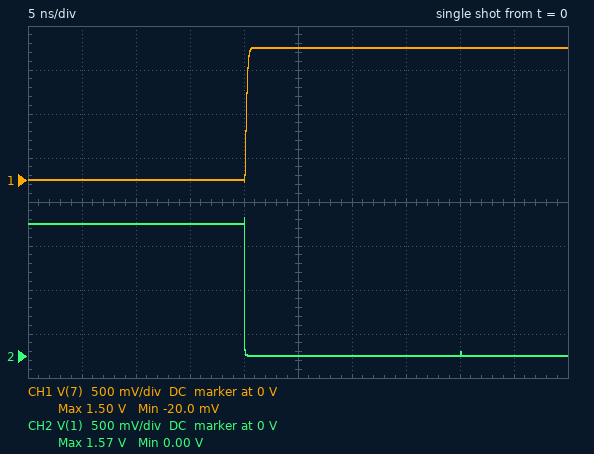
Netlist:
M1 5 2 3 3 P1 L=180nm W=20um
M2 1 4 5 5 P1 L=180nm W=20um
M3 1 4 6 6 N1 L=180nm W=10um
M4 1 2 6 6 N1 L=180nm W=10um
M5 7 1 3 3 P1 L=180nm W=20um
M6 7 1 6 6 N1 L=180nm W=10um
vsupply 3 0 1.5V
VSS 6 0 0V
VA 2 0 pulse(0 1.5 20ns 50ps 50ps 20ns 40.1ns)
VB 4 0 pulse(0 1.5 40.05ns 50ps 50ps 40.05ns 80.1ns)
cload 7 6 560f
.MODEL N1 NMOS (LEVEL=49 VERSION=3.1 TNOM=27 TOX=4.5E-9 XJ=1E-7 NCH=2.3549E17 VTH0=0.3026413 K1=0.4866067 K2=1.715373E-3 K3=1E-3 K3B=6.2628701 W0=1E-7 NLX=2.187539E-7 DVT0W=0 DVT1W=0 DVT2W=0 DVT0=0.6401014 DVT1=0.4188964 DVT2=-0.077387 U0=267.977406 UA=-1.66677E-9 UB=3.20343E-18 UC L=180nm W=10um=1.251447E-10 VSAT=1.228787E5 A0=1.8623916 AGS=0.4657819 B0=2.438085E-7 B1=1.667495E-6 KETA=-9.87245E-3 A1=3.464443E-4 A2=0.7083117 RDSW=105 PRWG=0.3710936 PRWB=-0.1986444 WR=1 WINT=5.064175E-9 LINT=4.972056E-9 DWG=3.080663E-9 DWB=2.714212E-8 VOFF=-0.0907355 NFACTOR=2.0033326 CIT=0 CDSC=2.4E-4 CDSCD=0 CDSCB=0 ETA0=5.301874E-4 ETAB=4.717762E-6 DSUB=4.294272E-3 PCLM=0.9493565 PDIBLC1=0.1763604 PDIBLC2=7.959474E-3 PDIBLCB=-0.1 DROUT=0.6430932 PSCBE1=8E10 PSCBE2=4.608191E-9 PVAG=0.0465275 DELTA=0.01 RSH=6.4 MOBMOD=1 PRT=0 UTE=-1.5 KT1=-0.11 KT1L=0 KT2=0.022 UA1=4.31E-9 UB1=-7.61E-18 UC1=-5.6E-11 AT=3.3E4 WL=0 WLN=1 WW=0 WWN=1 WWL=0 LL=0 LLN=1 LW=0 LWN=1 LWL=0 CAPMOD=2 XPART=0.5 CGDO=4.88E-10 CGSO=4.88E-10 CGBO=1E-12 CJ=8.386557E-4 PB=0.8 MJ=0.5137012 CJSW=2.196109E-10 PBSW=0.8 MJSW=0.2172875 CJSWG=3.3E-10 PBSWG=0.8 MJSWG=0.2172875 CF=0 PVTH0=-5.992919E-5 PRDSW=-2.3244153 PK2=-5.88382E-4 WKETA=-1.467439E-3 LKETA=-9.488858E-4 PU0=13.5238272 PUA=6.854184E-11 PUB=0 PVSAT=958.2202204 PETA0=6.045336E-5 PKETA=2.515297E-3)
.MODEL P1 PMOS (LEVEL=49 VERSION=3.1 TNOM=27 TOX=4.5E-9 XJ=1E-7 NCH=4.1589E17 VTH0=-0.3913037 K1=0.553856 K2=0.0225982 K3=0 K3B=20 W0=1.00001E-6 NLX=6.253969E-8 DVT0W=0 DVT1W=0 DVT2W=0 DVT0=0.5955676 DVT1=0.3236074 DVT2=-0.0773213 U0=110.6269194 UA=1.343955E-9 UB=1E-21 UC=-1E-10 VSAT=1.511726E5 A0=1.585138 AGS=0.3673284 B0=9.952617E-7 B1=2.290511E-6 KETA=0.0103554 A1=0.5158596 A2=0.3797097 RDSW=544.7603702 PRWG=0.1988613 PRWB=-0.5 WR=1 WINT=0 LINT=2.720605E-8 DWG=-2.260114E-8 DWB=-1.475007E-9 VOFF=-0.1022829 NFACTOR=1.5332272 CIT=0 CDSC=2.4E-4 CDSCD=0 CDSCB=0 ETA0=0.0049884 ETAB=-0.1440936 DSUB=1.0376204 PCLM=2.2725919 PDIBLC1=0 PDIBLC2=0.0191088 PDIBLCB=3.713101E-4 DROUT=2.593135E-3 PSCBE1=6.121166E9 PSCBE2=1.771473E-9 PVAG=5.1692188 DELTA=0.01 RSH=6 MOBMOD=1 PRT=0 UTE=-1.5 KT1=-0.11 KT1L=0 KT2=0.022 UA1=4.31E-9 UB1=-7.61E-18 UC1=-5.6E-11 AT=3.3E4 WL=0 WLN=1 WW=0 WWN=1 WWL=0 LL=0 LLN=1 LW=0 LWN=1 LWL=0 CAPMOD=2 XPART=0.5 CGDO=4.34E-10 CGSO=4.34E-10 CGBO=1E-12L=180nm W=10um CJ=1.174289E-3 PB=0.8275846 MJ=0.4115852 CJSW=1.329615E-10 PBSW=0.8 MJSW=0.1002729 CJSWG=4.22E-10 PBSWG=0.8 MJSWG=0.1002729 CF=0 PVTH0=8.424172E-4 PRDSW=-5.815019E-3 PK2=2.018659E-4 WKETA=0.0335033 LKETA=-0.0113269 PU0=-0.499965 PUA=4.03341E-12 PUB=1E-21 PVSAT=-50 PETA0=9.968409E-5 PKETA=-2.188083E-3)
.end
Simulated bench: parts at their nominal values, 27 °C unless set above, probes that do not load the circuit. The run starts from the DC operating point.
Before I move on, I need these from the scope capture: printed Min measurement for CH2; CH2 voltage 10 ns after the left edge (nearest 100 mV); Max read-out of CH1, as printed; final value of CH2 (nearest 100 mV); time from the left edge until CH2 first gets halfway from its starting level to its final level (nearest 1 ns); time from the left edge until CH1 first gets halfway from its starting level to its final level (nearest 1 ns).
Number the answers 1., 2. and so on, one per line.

1. 0.00 V
2. 1.5 V
3. 1.50 V
4. 0 V
5. 20 ns
6. 20 ns
